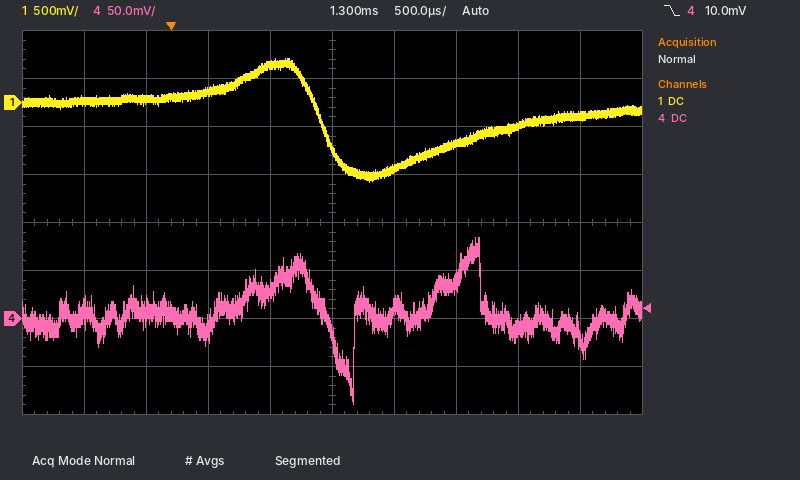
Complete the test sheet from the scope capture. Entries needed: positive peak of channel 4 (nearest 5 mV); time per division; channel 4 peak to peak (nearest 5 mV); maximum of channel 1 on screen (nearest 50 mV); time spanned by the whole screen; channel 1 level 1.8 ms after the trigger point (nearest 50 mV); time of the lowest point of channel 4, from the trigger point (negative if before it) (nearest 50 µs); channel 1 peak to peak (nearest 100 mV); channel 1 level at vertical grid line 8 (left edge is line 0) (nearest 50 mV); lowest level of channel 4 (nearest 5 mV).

85 mV
500 µs
175 mV
450 mV
5 ms
-700 mV
+1.45 ms
1.30 V
-250 mV
-90 mV
